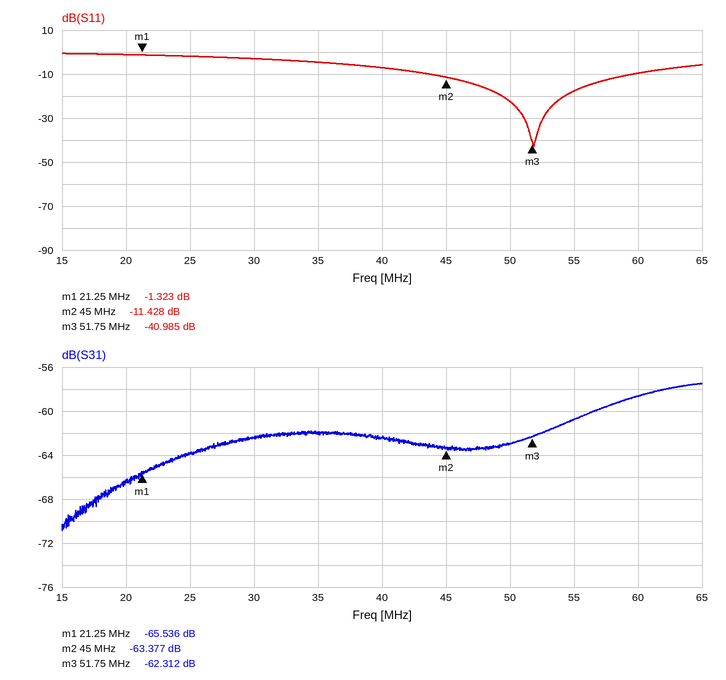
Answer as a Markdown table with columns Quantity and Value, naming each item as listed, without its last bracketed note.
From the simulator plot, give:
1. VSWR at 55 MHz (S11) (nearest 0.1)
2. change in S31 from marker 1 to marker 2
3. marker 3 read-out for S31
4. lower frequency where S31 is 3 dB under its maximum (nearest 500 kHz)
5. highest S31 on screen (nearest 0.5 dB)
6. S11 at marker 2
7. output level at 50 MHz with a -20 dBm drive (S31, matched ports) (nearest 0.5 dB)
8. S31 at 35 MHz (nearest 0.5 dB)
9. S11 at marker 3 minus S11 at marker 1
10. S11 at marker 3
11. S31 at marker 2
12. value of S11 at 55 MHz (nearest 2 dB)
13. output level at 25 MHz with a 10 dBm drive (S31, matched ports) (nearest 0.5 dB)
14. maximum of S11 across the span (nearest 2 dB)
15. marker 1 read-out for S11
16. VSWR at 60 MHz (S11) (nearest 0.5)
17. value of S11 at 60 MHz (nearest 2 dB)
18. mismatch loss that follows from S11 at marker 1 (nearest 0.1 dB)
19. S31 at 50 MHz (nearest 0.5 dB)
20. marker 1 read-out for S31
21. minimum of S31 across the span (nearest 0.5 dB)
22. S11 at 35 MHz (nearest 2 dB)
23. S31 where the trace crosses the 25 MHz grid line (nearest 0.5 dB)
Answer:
| Quantity | Value |
|---|---|
| VSWR at 55 MHz (S11) | 1.3 |
| change in S31 from marker 1 to marker 2 | 2.159 dB |
| marker 3 read-out for S31 | -62.312 dB |
| lower frequency where S31 is 3 dB under its maximum | 55.5 MHz |
| highest S31 on screen | -57.5 dB |
| S11 at marker 2 | -11.428 dB |
| output level at 50 MHz with a -20 dBm drive (S31, matched ports) | -83.0 dBm |
| S31 at 35 MHz | -62.0 dB |
| S11 at marker 3 minus S11 at marker 1 | -39.662 dB |
| S11 at marker 3 | -40.985 dB |
| S31 at marker 2 | -63.377 dB |
| value of S11 at 55 MHz | -18 dB |
| output level at 25 MHz with a 10 dBm drive (S31, matched ports) | -54.0 dBm |
| maximum of S11 across the span | 0 dB |
| marker 1 read-out for S11 | -1.323 dB |
| VSWR at 60 MHz (S11) | 2.0 |
| value of S11 at 60 MHz | -10 dB |
| mismatch loss that follows from S11 at marker 1 | 5.8 dB |
| S31 at 50 MHz | -63.0 dB |
| marker 1 read-out for S31 | -65.536 dB |
| minimum of S31 across the span | -71.0 dB |
| S11 at 35 MHz | -4 dB |
| S31 where the trace crosses the 25 MHz grid line | -64.0 dB |
